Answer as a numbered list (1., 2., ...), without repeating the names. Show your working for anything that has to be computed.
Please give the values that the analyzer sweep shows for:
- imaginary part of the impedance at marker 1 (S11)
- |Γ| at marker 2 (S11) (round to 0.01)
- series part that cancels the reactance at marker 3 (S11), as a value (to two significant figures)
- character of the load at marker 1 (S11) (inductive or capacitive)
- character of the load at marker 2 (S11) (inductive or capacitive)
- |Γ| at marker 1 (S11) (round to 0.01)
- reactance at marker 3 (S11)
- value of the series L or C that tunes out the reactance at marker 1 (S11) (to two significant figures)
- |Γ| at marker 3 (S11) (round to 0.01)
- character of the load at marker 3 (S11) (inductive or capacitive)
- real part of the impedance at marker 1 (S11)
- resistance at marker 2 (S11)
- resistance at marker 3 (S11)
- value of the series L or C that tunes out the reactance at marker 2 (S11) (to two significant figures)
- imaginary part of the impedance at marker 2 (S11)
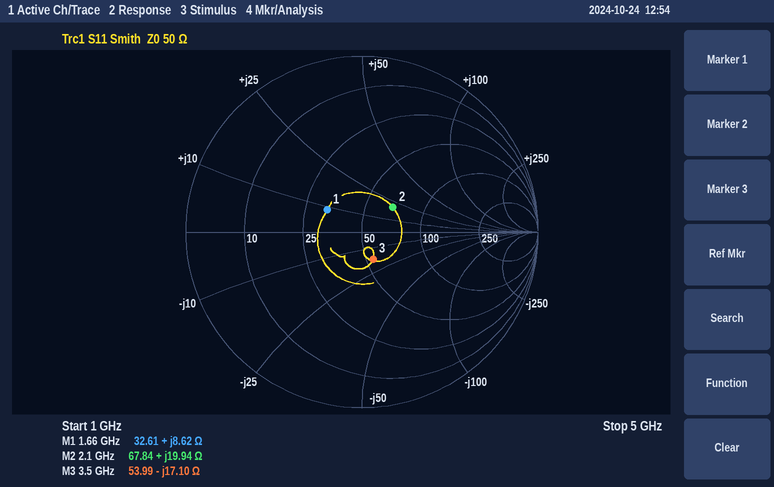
1. +8.62 Ω
2. 0.22
3. L = 17.1 Ω/(2π × 3.5 GHz) ≈ 778 pH, so 780 pH to two significant figures
4. inductive
5. inductive
6. 0.23
7. -17.10 Ω
8. C = 1/(2π × 1.66 GHz × 8.62 Ω) ≈ 11 pF
9. 0.17
10. capacitive
11. 32.61 Ω
12. 67.84 Ω
13. 53.99 Ω
14. C = 1/(2π × 2.1 GHz × 19.94 Ω) ≈ 3.8 pF
15. +19.94 Ω
